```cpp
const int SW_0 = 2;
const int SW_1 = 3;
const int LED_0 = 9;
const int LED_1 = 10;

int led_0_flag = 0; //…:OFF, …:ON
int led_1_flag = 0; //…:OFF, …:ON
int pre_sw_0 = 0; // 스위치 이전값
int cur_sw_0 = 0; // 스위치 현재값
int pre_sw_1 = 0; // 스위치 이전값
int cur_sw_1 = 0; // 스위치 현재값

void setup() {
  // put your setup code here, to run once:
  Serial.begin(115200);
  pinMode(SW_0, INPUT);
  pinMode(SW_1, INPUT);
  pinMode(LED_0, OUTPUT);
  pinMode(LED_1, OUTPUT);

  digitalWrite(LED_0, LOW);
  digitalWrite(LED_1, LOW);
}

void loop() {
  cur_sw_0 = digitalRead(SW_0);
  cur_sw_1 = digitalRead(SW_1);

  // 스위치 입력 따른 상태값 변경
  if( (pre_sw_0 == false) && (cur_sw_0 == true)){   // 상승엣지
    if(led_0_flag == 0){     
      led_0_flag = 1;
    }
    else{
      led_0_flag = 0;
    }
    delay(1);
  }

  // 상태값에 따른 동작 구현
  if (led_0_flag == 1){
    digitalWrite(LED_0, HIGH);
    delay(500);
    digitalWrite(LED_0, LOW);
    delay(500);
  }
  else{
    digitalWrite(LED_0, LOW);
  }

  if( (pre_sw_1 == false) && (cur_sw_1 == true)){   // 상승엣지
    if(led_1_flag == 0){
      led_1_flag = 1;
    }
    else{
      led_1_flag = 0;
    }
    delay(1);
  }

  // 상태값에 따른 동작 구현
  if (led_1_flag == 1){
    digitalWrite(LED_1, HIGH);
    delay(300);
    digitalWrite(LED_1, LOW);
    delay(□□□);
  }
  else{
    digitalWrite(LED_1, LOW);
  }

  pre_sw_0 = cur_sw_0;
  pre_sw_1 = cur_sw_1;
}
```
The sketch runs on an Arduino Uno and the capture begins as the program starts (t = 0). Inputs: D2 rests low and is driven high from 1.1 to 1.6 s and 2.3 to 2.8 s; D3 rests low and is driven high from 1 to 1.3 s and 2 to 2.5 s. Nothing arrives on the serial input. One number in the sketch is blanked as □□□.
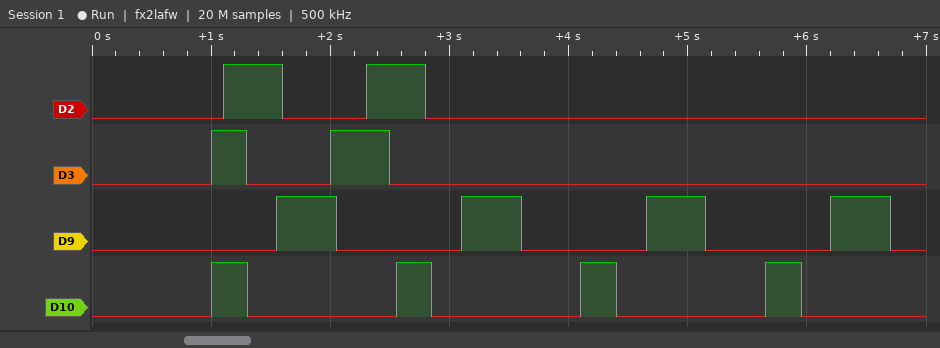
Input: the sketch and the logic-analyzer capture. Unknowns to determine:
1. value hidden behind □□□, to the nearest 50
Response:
250
